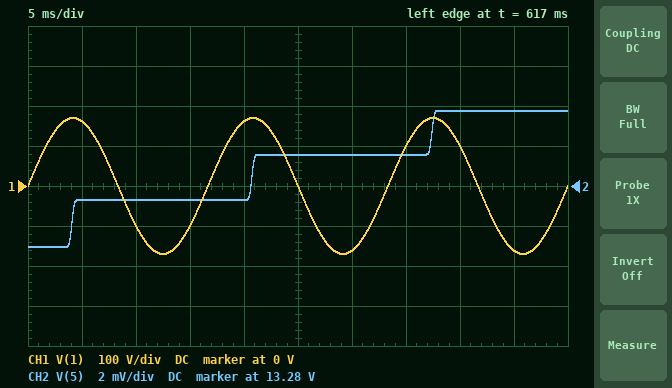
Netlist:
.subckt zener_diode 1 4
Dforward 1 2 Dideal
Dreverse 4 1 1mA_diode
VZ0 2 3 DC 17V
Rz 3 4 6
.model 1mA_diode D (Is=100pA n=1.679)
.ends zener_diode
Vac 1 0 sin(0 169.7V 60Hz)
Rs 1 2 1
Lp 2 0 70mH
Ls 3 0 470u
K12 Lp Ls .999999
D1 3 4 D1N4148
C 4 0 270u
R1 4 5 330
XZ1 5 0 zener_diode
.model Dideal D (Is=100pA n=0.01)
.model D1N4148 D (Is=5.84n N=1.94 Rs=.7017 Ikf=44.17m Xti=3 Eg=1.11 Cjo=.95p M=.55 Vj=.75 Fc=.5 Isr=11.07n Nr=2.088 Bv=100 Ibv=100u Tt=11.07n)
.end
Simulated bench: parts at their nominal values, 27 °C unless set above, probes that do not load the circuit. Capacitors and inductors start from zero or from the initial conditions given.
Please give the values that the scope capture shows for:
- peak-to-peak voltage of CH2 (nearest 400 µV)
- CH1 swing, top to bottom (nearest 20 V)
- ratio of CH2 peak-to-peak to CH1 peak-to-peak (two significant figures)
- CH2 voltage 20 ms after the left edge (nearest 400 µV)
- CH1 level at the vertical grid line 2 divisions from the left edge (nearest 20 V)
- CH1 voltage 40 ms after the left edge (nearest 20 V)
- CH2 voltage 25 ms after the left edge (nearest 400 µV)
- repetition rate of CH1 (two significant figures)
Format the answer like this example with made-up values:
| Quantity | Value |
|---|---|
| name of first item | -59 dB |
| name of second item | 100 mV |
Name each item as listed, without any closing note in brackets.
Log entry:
| Quantity | Value |
|---|---|
| peak-to-peak voltage of CH2 | 6.8 mV |
| CH1 swing, top to bottom | 340 V |
| ratio of CH2 peak-to-peak to CH1 peak-to-peak | 0.000020 |
| CH2 voltage 20 ms after the left edge | 13.2752 V |
| CH1 level at the vertical grid line 2 divisions from the left edge | -100 V |
| CH1 voltage 40 ms after the left edge | 100 V |
| CH2 voltage 25 ms after the left edge | 13.2776 V |
| repetition rate of CH1 | 60 Hz |
